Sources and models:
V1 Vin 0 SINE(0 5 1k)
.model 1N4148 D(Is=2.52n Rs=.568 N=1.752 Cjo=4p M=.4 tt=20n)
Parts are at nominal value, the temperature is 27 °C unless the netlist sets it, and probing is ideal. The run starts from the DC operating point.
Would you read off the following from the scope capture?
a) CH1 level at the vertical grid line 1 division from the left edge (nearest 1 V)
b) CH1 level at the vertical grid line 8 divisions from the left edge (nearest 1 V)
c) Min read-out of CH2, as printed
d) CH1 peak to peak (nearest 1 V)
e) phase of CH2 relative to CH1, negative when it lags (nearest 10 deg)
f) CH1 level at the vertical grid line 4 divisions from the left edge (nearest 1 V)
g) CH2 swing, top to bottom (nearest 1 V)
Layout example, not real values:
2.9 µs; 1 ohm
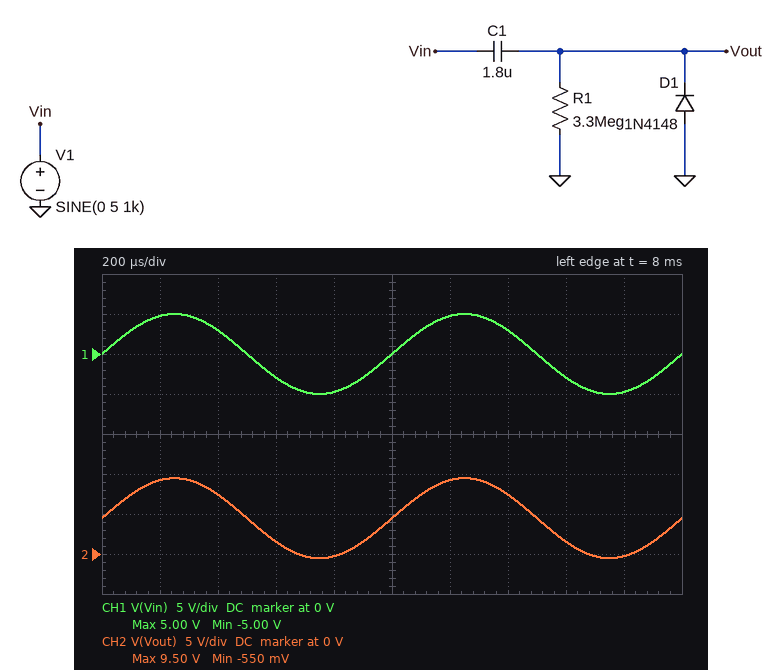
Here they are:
5 V; -3 V; -550 mV; 10 V; 0 deg; -5 V; 10 V
